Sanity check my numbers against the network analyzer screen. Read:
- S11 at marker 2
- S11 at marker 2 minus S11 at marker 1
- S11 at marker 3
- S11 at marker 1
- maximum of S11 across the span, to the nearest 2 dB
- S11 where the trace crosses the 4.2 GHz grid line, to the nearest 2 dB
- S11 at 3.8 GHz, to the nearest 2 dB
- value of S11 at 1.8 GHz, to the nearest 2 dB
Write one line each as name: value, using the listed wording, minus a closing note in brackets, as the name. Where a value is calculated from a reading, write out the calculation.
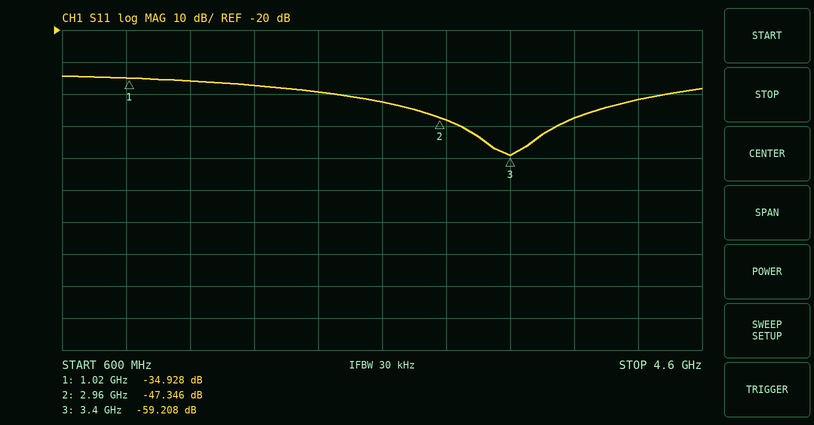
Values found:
S11 at marker 2: -47.346 dB
S11 at marker 2 minus S11 at marker 1: -47.346 − (-34.928) = -12.418 dB
S11 at marker 3: -59.208 dB
S11 at marker 1: -34.928 dB
maximum of S11 across the span, to the nearest 2 dB: -34 dB
S11 where the trace crosses the 4.2 GHz grid line, to the nearest 2 dB: -42 dB
S11 at 3.8 GHz, to the nearest 2 dB: -48 dB
value of S11 at 1.8 GHz, to the nearest 2 dB: -38 dB
